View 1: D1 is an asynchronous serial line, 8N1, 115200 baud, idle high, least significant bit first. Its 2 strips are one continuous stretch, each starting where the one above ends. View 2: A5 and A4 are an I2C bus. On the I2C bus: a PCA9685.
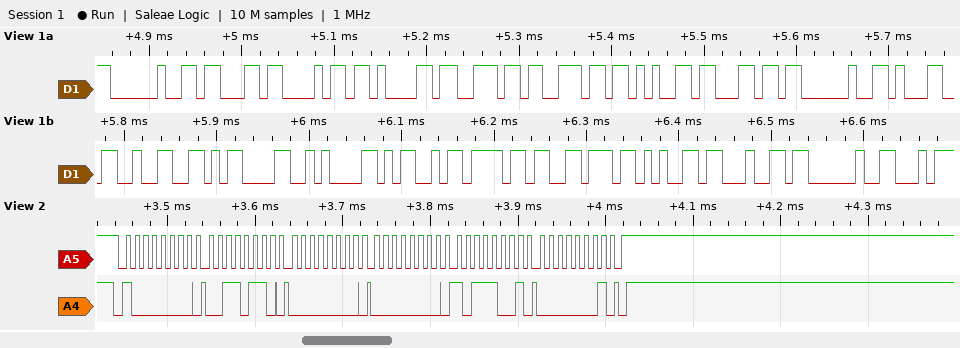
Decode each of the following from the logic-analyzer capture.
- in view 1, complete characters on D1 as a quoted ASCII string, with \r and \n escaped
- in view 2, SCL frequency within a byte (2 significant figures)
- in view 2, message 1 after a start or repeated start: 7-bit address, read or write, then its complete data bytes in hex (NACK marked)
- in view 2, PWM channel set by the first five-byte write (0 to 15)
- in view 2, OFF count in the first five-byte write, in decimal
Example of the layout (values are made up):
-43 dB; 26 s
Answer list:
" channel 12\r\nMoved "; 100 kHz; 0x40 write: 36 00 00 B9 01; 12; 441
